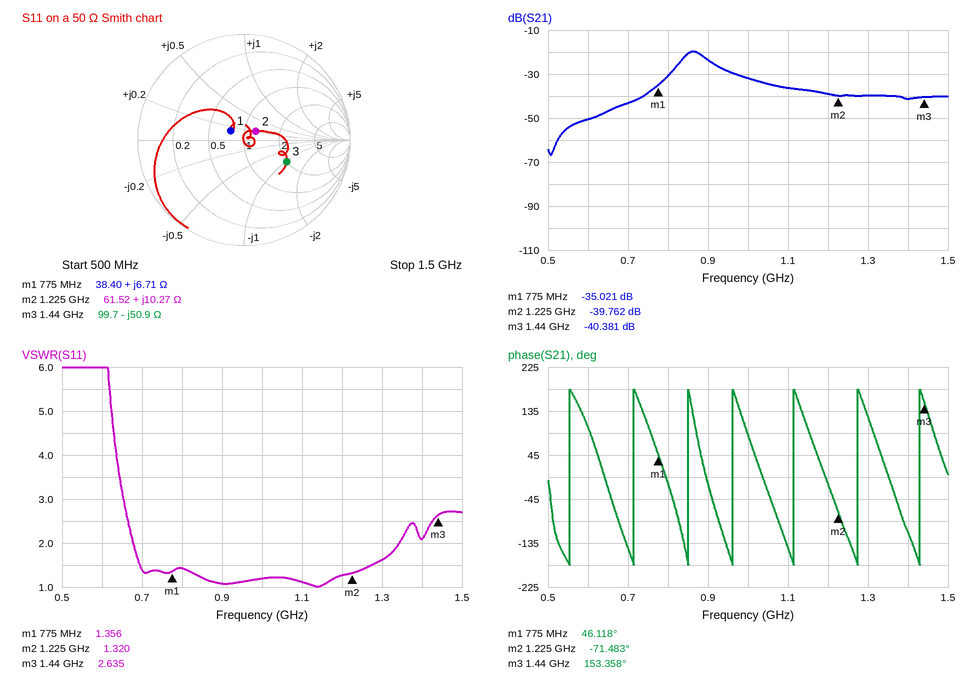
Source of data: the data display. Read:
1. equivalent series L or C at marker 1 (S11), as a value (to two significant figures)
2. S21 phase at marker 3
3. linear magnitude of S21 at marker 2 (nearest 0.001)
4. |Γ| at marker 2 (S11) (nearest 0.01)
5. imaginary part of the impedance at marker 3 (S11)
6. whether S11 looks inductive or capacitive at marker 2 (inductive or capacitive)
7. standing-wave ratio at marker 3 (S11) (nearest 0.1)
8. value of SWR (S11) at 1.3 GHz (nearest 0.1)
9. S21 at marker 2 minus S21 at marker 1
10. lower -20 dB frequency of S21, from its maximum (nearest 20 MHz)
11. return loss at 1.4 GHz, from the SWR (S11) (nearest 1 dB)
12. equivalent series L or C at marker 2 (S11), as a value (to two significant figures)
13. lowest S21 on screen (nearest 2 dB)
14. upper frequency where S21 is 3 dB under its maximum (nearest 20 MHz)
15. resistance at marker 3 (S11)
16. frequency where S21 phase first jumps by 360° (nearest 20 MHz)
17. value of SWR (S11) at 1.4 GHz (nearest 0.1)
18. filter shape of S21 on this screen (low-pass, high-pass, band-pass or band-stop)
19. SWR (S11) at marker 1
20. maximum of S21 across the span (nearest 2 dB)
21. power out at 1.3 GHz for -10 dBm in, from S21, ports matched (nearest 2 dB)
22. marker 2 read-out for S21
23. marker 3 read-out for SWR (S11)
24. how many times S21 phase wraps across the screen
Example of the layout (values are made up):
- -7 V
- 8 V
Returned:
- 1.4 nH
- 153.358°
- 0.010
- 0.14
- -50.9 Ω
- inductive
- 2.6
- 1.6
- -4.741 dB
- 740 MHz
- 9 dB
- 1.3 nH
- -66 dB
- 900 MHz
- 99.7 Ω
- 560 MHz
- 2.1
- band-pass
- 1.356
- -20 dB
- -50 dBm
- -39.762 dB
- 2.635
- 7
